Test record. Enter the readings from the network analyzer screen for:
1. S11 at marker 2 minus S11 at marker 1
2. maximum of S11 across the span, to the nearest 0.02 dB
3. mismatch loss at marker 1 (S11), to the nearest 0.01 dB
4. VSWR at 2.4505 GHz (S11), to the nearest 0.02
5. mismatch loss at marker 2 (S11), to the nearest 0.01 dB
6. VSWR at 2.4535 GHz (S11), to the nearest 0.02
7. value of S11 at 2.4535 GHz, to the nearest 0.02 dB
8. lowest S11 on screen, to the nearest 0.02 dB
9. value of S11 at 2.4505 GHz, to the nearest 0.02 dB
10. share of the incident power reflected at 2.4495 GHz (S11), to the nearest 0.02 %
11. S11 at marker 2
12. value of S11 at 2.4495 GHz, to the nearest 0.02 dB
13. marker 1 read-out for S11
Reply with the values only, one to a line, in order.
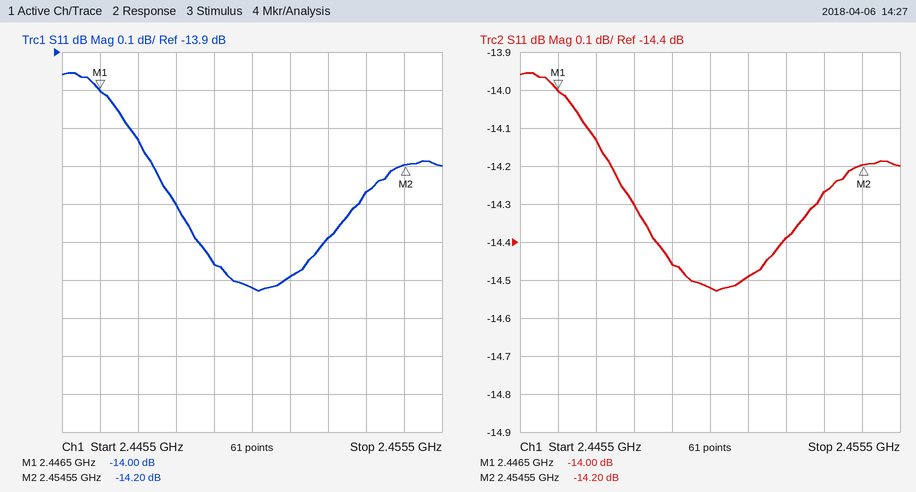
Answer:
-0.20 dB
-13.96 dB
0.18 dB
1.46
0.17 dB
1.48
-14.26 dB
-14.52 dB
-14.52 dB
3.58 %
-14.20 dB
-14.46 dB
-14.00 dB
